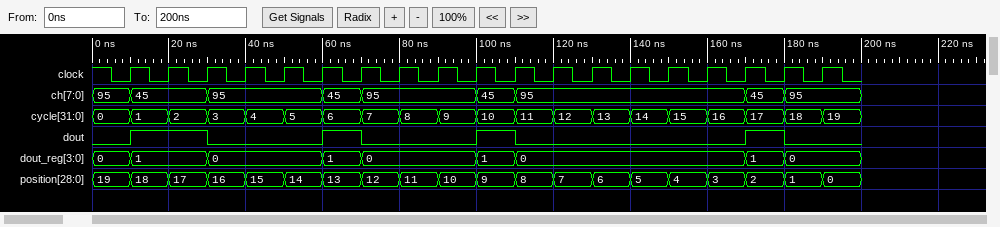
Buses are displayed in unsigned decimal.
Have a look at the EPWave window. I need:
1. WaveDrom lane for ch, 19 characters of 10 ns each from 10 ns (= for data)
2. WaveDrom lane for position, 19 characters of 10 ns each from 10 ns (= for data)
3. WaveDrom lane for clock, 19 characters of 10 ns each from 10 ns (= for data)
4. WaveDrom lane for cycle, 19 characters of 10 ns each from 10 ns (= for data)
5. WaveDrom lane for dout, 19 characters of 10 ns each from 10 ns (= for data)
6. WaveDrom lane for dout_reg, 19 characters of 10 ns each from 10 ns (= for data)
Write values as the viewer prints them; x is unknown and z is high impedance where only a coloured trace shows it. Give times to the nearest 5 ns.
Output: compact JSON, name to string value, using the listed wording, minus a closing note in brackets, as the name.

{"WaveDrom lane for ch, 19 characters of 10 ns each from 10 ns": "{name: 'ch', wave: '=.=..==..==.....==.', data: '45 95 45 95 45 95 45 95'}", "WaveDrom lane for position, 19 characters of 10 ns each from 10 ns": "{name: 'position', wave: '===================', data: '18 17 16 15 14 13 12 11 10 9 8 7 6 5 4 3 2 1 0'}", "WaveDrom lane for clock, 19 characters of 10 ns each from 10 ns": "{name: 'clock', wave: 'p..................'}", "WaveDrom lane for cycle, 19 characters of 10 ns each from 10 ns": "{name: 'cycle', wave: '===================', data: '1 2 3 4 5 6 7 8 9 10 11 12 13 14 15 16 17 18 19'}", "WaveDrom lane for dout, 19 characters of 10 ns each from 10 ns": "{name: 'dout', wave: '1.0..10..10.....10.'}", "WaveDrom lane for dout_reg, 19 characters of 10 ns each from 10 ns": "{name: 'dout_reg', wave: '=.=..==..==.....==.', data: '1 0 1 0 1 0 1 0'}"}
